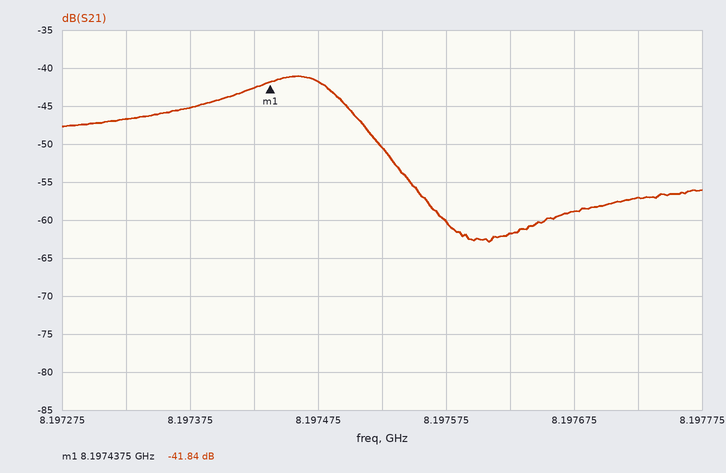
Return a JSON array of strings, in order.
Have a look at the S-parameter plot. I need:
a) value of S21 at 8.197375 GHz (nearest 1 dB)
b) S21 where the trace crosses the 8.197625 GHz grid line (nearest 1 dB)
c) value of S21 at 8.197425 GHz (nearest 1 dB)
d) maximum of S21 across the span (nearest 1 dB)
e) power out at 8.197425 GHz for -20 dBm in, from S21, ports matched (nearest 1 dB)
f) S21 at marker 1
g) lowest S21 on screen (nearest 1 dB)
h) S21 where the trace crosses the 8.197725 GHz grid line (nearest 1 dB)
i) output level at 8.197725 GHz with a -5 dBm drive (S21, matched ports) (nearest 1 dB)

["-45 dB", "-62 dB", "-43 dB", "-41 dB", "-63 dBm", "-41.84 dB", "-63 dB", "-57 dB", "-62 dBm"]
